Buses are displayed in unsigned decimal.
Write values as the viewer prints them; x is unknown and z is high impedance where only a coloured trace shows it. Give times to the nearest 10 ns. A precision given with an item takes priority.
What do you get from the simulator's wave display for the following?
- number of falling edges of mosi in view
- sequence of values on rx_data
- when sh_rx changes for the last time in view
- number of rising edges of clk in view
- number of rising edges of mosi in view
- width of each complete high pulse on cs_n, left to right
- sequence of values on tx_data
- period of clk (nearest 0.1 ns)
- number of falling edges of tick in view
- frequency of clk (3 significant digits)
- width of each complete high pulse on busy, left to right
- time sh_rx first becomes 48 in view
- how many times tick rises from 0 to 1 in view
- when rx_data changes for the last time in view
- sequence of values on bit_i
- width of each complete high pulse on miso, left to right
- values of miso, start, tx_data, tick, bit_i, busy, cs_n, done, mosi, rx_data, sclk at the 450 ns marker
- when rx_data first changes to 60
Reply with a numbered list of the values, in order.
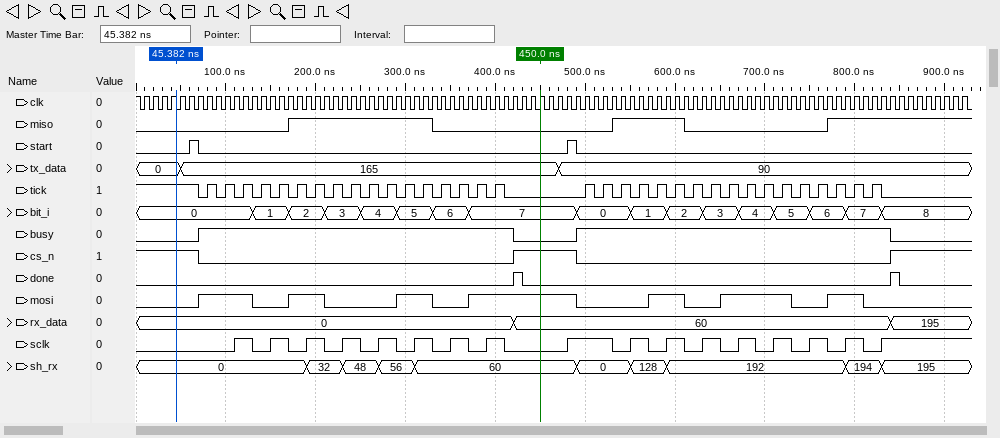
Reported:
1. 7
2. 0, 60, 195
3. 830 ns
4. 92
5. 7
6. 70 ns
7. 0, 165, 90
8. 10 ns
9. 35
10. 100 MHz
11. 350 ns, 350 ns
12. 230 ns
13. 34
14. 840 ns
15. 0, 1, 2, 3, 4, 5, 6, 7, 0, 1, 2, 3, 4, 5, 6, 7, 8
16. 160 ns, 80 ns
17. miso=0, start=0, tx_data=165, tick=0, bit_i=7, busy=0, cs_n=1, done=0, mosi=1, rx_data=60, sclk=0
18. 420 ns
